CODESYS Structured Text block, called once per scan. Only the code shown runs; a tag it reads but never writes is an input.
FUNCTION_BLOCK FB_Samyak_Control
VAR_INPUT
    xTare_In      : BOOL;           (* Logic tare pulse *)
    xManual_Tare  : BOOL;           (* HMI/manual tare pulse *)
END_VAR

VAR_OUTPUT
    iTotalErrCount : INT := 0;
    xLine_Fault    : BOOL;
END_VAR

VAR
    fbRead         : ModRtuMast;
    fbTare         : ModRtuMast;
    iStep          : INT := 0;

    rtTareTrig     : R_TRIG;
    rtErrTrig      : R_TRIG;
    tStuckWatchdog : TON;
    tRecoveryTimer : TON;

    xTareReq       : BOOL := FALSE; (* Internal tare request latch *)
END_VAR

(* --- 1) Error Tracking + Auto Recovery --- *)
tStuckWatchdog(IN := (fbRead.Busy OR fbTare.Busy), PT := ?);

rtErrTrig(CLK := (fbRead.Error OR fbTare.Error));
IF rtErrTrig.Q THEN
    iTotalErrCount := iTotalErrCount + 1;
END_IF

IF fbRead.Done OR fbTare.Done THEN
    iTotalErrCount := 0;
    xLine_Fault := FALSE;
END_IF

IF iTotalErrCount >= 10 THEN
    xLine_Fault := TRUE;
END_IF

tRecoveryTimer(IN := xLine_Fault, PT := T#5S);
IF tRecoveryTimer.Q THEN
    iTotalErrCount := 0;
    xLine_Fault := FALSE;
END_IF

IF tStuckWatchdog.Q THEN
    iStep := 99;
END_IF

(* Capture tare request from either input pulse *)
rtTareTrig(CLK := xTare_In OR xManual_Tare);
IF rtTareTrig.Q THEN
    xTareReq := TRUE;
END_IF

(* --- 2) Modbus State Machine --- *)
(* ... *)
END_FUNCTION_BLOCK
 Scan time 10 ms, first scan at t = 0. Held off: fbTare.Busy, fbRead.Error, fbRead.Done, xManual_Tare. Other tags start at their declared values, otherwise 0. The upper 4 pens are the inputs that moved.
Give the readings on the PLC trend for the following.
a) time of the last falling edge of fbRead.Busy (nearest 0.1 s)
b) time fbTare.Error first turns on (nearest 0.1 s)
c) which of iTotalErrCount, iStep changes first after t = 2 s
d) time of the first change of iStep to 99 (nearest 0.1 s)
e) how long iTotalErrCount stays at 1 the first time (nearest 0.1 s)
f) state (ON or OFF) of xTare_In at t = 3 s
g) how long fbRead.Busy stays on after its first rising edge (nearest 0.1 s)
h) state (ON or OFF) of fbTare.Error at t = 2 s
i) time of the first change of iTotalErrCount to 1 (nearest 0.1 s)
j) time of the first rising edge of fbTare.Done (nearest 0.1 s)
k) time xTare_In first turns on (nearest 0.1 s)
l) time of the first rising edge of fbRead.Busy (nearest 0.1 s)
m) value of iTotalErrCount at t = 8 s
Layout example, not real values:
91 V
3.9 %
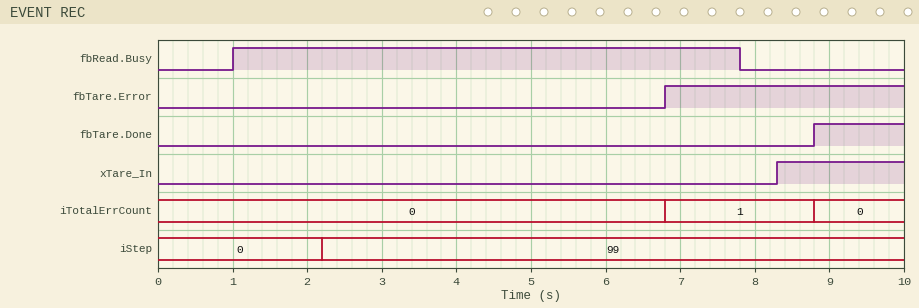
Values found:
7.8 s
6.8 s
iStep
2.2 s
2.0 s
OFF
6.8 s
OFF
6.8 s
8.8 s
8.3 s
1.0 s
1
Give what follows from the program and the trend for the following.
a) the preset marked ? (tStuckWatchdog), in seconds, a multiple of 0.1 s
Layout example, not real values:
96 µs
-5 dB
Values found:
1.2 s
